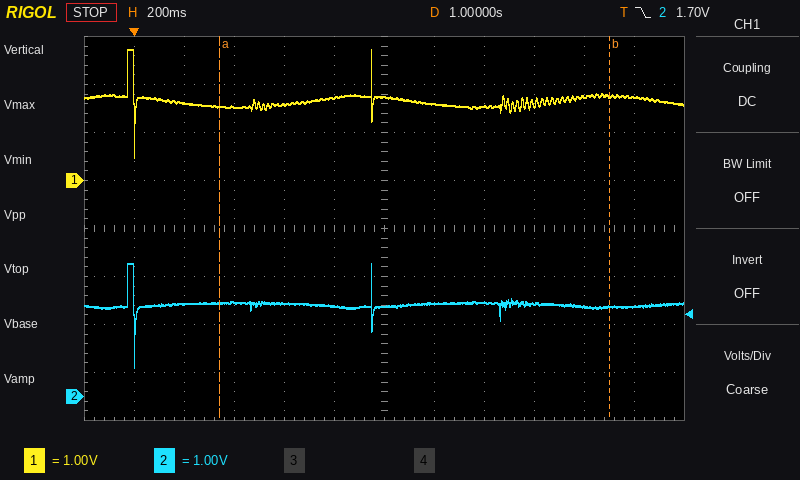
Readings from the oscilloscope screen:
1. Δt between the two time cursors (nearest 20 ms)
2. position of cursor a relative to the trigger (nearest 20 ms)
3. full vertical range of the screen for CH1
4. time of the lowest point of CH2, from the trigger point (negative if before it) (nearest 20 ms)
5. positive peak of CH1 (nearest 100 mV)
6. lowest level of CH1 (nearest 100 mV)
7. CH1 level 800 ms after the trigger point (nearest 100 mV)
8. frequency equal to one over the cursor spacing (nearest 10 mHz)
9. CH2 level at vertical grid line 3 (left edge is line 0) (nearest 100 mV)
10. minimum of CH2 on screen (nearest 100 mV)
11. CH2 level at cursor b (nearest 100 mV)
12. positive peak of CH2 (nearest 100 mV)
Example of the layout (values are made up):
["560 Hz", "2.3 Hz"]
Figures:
["1.56 s", "+340 ms", "8 V", "0 ms", "2.7 V", "500 mV", "1.7 V", "640 mHz", "2.0 V", "600 mV", "1.9 V", "2.8 V"]
